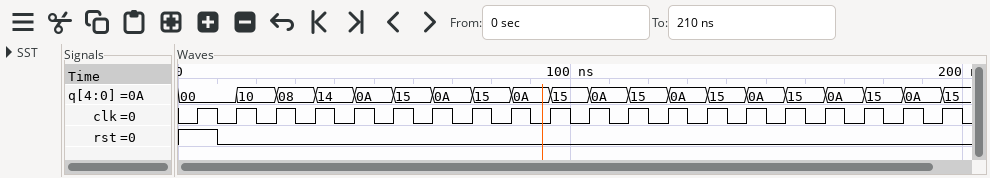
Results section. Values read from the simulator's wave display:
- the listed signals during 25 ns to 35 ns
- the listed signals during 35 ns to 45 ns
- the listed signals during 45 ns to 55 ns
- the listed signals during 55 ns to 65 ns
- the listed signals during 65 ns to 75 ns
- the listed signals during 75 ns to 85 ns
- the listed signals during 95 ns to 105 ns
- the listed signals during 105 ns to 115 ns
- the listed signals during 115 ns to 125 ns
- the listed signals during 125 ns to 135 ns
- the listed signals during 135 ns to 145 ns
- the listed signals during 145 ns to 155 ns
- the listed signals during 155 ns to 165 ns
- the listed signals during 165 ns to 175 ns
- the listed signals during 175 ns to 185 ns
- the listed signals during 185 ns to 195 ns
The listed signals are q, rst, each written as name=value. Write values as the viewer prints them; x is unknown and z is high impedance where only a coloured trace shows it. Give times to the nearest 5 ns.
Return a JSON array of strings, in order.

["q=08, rst=0", "q=14, rst=0", "q=0A, rst=0", "q=15, rst=0", "q=0A, rst=0", "q=15, rst=0", "q=15, rst=0", "q=0A, rst=0", "q=15, rst=0", "q=0A, rst=0", "q=15, rst=0", "q=0A, rst=0", "q=15, rst=0", "q=0A, rst=0", "q=15, rst=0", "q=0A, rst=0"]
